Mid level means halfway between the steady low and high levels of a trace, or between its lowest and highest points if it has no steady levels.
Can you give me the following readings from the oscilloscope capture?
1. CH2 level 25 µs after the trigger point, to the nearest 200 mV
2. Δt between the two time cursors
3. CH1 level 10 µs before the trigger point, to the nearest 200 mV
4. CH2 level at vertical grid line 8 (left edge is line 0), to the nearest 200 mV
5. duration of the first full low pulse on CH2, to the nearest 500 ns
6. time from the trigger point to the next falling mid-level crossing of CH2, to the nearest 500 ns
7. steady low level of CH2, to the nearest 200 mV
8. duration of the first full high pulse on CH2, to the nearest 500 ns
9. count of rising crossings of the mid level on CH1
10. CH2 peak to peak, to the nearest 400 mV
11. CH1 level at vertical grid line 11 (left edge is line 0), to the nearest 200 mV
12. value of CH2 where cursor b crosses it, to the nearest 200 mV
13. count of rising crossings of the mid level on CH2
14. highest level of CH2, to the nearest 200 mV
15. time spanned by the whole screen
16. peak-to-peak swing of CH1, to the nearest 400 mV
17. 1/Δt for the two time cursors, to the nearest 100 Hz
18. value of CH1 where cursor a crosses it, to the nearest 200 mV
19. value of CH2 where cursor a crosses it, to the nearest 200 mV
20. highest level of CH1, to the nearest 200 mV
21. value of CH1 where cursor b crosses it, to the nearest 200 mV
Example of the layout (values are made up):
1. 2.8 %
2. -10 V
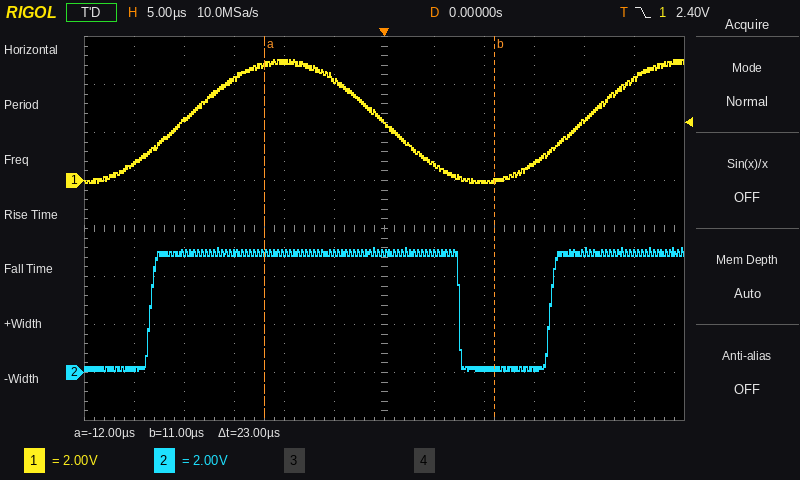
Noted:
1. 5.0 V
2. 23 µs
3. 5.0 V
4. 200 mV
5. 9.0 µs
6. 7.5 µs
7. 200 mV
8. 31.0 µs
9. 2
10. 5.2 V
11. 4.2 V
12. 200 mV
13. 2
14. 5.2 V
15. 60 µs
16. 5.2 V
17. 43.5 kHz
18. 4.8 V
19. 5.0 V
20. 5.0 V
21. 0.0 V
